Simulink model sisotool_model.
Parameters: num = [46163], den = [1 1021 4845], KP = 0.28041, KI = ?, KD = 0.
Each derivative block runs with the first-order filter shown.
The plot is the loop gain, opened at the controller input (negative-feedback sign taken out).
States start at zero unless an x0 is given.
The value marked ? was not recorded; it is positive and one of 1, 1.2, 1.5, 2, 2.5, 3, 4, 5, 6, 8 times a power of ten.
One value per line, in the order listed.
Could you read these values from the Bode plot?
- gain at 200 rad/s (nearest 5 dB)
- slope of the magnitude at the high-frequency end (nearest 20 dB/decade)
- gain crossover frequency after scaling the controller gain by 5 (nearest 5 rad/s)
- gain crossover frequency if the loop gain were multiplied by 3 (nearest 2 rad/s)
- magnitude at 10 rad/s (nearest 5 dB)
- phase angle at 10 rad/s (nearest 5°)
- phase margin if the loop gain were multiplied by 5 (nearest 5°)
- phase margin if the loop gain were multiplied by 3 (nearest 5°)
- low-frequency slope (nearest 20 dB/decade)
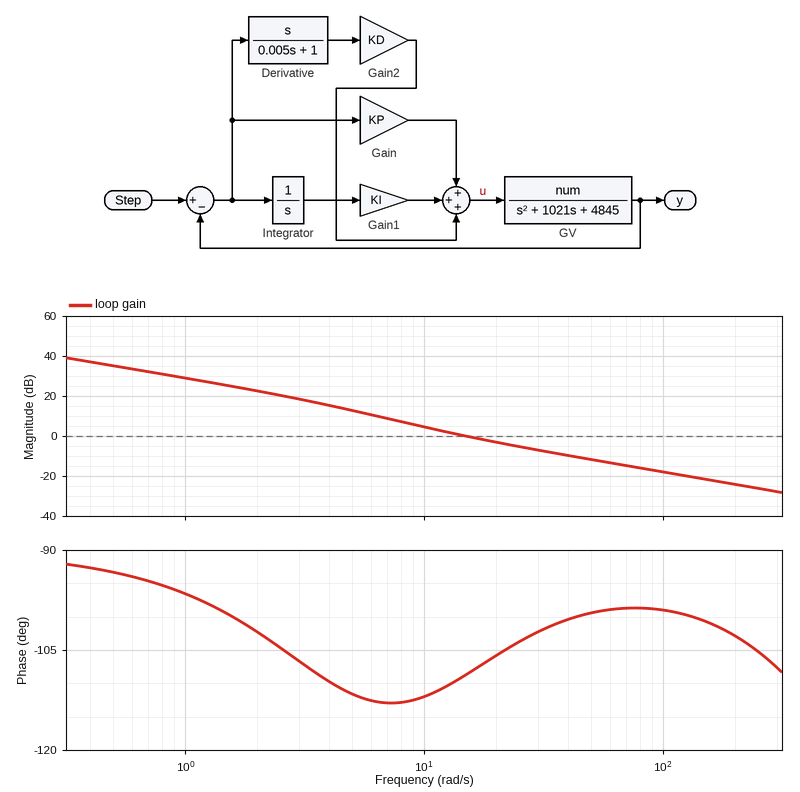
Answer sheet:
-25 dB
-20 dB/decade
65 rad/s
40 rad/s
5 dB
-110°
80°
80°
-20 dB/decade
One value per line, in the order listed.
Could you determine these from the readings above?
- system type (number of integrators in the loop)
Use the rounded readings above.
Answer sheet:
1
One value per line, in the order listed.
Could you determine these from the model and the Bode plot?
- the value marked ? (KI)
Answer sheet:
3
